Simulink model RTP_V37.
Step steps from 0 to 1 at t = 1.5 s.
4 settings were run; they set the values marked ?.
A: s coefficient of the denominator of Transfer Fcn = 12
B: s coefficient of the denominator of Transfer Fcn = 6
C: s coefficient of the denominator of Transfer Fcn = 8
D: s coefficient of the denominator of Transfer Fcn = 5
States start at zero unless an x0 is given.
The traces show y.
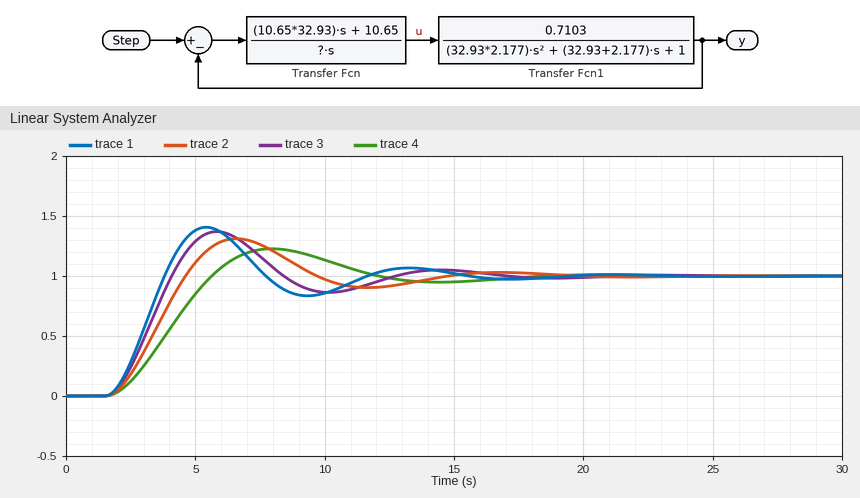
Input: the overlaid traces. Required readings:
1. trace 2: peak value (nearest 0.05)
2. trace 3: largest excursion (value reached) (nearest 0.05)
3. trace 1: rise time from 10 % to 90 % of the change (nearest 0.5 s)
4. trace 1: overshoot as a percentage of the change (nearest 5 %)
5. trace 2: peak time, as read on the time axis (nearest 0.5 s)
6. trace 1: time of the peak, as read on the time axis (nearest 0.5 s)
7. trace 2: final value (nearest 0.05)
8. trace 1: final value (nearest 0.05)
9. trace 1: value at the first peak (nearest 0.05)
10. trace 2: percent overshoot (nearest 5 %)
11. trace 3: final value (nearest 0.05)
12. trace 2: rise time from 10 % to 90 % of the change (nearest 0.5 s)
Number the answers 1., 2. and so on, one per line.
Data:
1. 1.30
2. 1.35
3. 1.5 s
4. 40 %
5. 6.5 s
6. 5.5 s
7. 1.00
8. 1.00
9. 1.40
10. 30 %
11. 1.00
12. 2.0 s
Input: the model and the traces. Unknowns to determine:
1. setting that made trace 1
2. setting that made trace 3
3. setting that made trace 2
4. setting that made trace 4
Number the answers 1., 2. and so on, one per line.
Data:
1. D
2. B
3. C
4. A
